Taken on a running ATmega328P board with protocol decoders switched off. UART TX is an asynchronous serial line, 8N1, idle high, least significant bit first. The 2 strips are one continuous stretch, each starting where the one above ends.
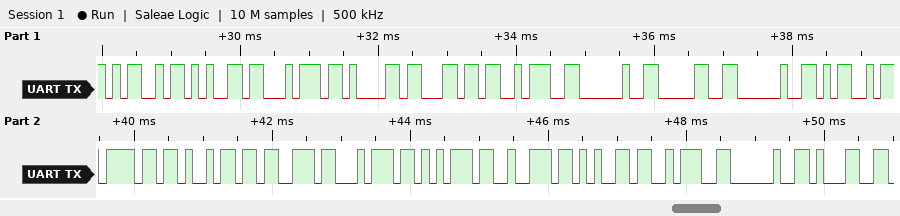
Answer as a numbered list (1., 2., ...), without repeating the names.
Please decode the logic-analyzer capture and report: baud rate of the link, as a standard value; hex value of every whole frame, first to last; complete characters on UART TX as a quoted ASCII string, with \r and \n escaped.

1. 9600 baud
2. 4D 65 74 61 6C 3A 20 30 20 4D 6F 69 73 74 75 72 65 3A 20 31
3. "Metal: 0 Moisture: 1"
